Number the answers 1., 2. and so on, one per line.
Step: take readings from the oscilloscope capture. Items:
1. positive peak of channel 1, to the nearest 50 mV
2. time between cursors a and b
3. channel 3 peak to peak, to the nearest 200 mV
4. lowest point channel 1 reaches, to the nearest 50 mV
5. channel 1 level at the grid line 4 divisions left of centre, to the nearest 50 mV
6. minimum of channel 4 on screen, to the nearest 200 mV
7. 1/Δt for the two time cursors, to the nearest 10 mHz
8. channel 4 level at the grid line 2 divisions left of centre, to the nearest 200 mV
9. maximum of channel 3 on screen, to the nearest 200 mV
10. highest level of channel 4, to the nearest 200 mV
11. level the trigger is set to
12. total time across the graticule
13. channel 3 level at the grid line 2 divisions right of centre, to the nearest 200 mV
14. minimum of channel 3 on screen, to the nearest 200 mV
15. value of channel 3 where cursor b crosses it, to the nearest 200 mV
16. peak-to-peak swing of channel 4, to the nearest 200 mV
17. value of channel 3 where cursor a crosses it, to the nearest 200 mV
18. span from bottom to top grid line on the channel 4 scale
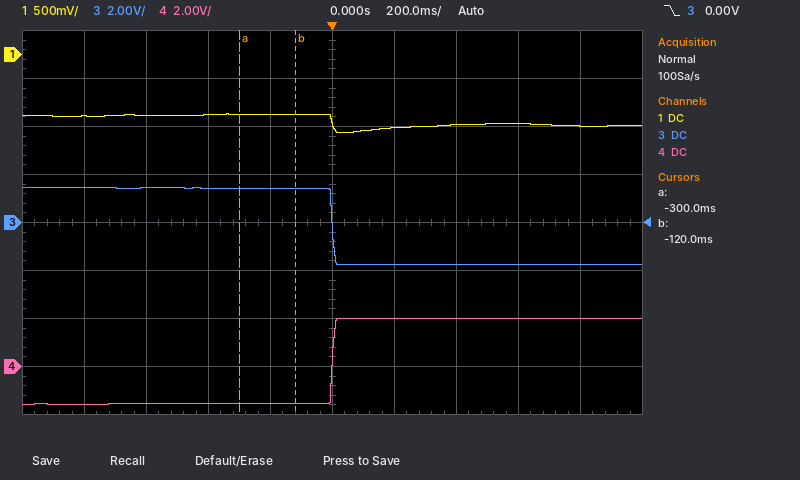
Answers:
1. -600 mV
2. 180 ms
3. 3.2 V
4. -800 mV
5. -650 mV
6. -1.6 V
7. 5.56 Hz
8. -1.6 V
9. 1.4 V
10. 2.0 V
11. 0.00 V
12. 2 s
13. -1.8 V
14. -1.8 V
15. 1.4 V
16. 3.6 V
17. 1.4 V
18. 16 V
